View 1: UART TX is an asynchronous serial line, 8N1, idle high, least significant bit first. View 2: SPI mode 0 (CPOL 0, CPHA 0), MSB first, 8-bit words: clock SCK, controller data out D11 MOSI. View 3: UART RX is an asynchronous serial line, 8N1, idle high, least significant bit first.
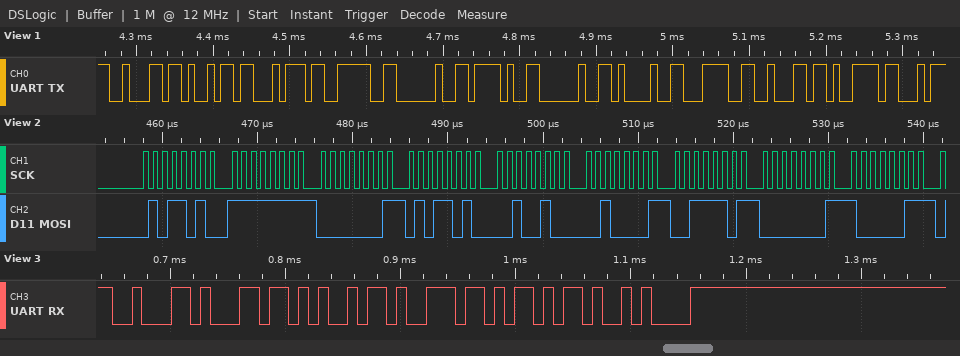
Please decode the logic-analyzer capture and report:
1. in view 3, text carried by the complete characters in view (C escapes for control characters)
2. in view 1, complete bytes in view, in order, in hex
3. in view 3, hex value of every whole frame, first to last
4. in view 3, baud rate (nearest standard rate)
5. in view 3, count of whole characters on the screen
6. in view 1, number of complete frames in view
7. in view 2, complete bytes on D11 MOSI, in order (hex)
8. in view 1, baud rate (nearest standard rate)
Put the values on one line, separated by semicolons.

"blink\n"; 0x62 0x69 0x74 0x3E 0x20 0x2F 0x20 0x21 0x3C 0x62 0x79; 0x62 0x6C 0x69 0x6E 0x6B 0x0A; 115200 baud; 6; 11; 0x5A 0xFF 0x01 0x5A 0x24 0x21 0x3D 0x01 0x83; 115200 baud
